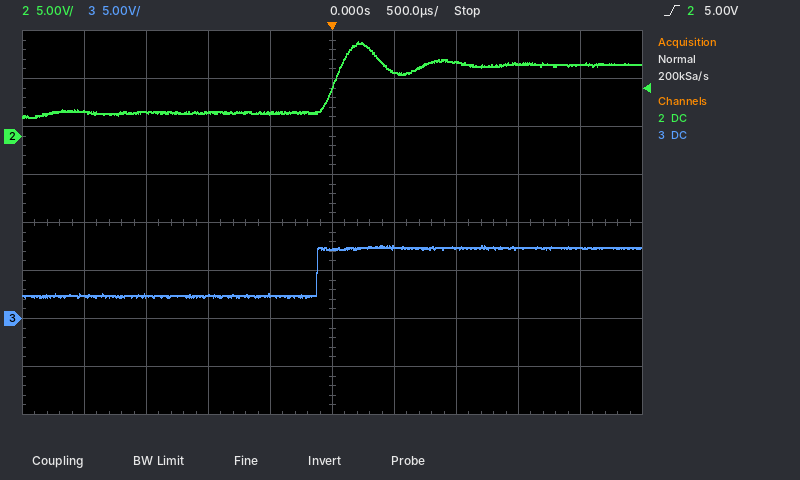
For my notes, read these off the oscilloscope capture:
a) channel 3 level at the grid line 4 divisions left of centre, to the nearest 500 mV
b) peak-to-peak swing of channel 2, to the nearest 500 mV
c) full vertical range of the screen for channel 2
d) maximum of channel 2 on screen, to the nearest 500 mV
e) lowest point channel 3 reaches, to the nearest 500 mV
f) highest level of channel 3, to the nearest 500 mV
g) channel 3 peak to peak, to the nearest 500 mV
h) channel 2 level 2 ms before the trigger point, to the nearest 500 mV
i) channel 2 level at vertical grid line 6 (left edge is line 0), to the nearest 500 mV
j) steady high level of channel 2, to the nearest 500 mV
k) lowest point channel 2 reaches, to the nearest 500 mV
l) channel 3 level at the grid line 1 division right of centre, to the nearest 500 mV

2.5 V
8.0 V
40 V
10.0 V
2.0 V
7.5 V
5.5 V
2.5 V
6.5 V
7.5 V
2.0 V
7.5 V
